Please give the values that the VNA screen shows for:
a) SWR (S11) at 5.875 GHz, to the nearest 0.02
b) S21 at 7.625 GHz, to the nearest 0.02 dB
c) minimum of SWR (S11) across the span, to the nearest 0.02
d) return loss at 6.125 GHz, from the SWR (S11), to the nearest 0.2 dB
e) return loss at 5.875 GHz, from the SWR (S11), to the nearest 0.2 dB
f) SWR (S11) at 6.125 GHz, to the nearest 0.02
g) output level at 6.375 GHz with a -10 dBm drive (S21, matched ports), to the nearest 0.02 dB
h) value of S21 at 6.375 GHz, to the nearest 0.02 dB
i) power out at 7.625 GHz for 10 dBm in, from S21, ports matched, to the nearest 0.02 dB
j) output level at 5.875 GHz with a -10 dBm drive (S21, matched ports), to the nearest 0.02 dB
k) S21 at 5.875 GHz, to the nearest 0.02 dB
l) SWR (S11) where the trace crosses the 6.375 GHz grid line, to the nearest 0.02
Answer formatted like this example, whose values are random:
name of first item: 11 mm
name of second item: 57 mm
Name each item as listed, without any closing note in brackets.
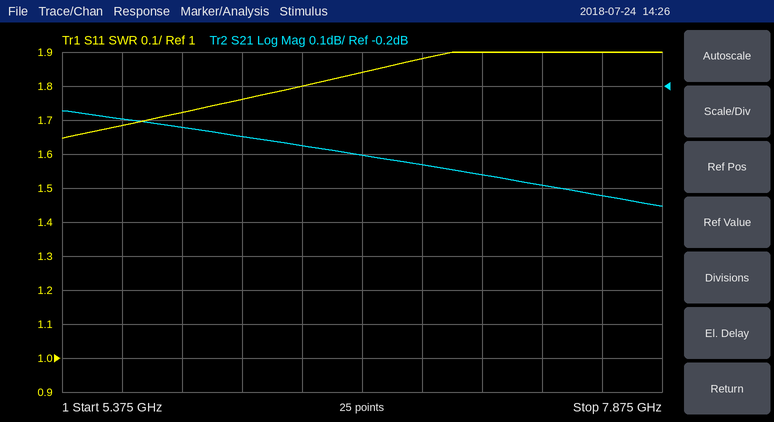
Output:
SWR (S11) at 5.875 GHz, to the nearest 0.02: 1.72
S21 at 7.625 GHz, to the nearest 0.02 dB: -0.52 dB
minimum of SWR (S11) across the span, to the nearest 0.02: 1.64
return loss at 6.125 GHz, from the SWR (S11), to the nearest 0.2 dB: 11.2 dB
return loss at 5.875 GHz, from the SWR (S11), to the nearest 0.2 dB: 11.6 dB
SWR (S11) at 6.125 GHz, to the nearest 0.02: 1.76
output level at 6.375 GHz with a -10 dBm drive (S21, matched ports), to the nearest 0.02 dB: -10.38 dBm
value of S21 at 6.375 GHz, to the nearest 0.02 dB: -0.38 dB
power out at 7.625 GHz for 10 dBm in, from S21, ports matched, to the nearest 0.02 dB: 9.48 dBm
output level at 5.875 GHz with a -10 dBm drive (S21, matched ports), to the nearest 0.02 dB: -10.32 dBm
S21 at 5.875 GHz, to the nearest 0.02 dB: -0.32 dB
SWR (S11) where the trace crosses the 6.375 GHz grid line, to the nearest 0.02: 1.80
